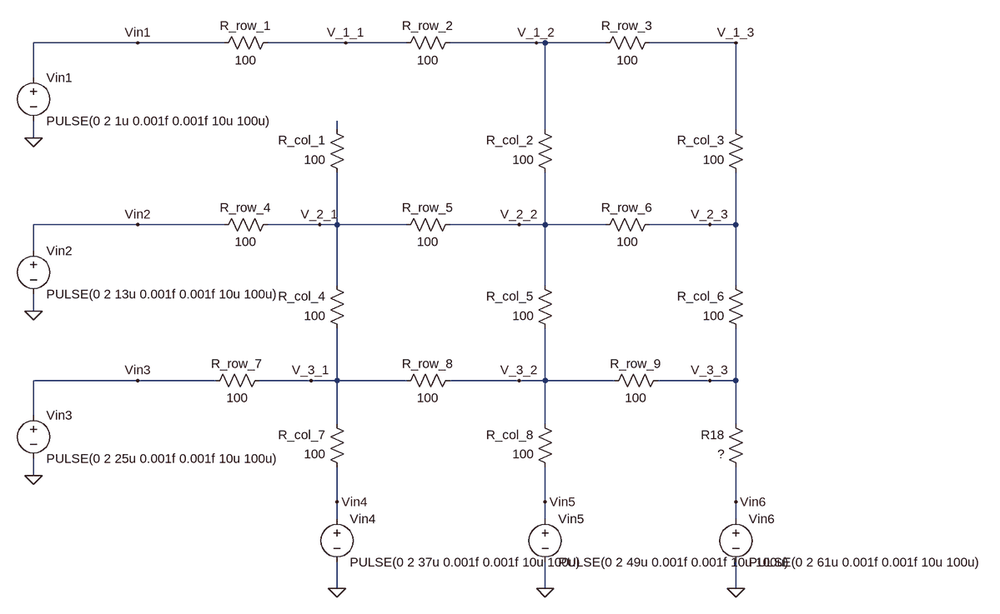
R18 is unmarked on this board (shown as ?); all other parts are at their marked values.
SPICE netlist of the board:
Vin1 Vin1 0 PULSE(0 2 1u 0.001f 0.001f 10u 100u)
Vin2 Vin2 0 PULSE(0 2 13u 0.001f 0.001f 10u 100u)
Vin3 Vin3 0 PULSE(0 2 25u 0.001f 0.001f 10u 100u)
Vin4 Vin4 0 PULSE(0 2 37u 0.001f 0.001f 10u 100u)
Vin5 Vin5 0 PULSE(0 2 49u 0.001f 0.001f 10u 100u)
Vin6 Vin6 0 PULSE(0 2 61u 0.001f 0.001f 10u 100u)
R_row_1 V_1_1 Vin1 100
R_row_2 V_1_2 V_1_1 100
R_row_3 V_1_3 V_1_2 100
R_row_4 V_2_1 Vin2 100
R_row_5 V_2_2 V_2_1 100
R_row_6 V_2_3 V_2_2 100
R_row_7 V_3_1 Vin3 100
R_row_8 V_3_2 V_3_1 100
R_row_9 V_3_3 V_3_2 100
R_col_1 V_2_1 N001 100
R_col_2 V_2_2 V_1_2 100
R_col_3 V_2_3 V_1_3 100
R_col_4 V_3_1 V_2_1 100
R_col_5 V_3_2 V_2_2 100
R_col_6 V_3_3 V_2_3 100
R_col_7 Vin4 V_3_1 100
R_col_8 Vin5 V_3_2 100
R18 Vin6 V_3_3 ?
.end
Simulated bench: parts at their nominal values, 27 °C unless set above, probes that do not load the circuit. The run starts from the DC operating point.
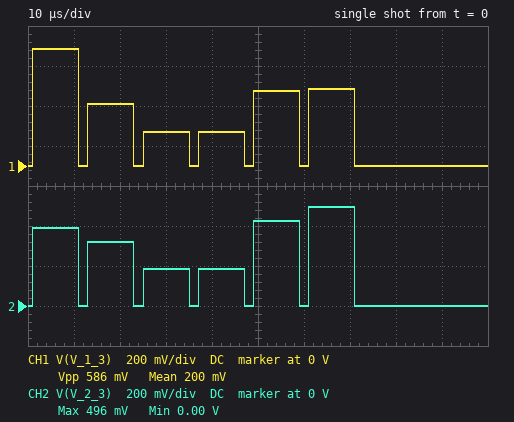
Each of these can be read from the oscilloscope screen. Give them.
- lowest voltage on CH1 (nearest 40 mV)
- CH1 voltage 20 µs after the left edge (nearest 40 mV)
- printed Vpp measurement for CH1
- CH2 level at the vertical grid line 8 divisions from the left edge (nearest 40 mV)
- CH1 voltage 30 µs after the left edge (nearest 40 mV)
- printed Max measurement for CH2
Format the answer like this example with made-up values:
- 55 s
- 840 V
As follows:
- 0 V
- 320 mV
- 586 mV
- 0 V
- 160 mV
- 496 mV
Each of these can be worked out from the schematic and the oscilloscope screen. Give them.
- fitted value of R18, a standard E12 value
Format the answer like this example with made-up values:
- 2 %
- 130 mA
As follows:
- 150 Ω
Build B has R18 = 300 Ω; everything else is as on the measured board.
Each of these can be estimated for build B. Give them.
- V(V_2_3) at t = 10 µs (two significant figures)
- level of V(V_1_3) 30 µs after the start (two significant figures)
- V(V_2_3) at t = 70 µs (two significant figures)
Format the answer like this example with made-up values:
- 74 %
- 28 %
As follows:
- 420 mV
- 190 mV
- 310 mV
